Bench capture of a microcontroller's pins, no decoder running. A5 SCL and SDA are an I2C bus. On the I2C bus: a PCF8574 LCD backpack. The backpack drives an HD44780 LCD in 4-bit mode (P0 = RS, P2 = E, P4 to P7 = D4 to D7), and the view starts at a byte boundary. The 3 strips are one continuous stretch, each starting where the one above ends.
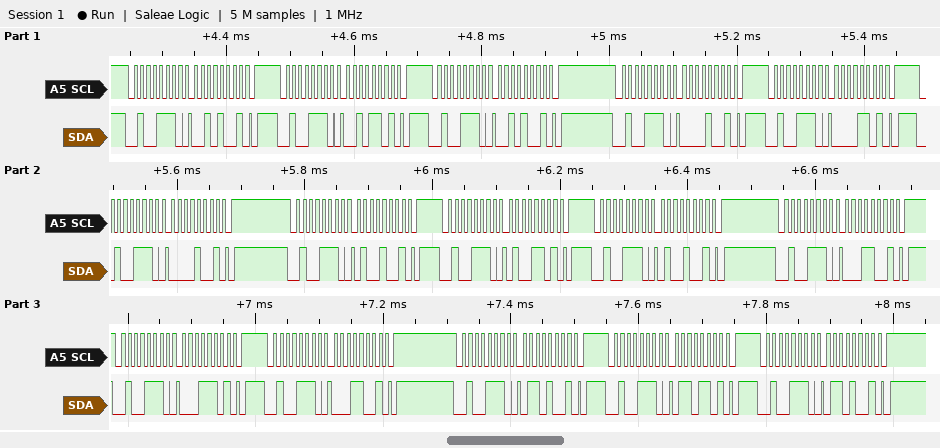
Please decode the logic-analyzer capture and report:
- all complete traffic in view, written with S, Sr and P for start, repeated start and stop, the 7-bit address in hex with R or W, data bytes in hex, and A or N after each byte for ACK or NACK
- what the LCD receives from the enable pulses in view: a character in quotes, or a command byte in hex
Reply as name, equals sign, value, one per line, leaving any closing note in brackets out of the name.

all complete traffic in view, written with S, Sr and P for start, repeated start and stop, the 7-bit address in hex with R or W, data bytes in hex, and A or N after each byte for ACK or NACK = S 27W A 29 A P S 27W A 2D A P S 27W A 29 A P S 27W A 09 A P S 27W A 0D A P S 27W A 09 A P S 27W A 49 A P S 27W A 4D A P S 27W A 49 A P S 27W A 19 A P S 27W A 1D A P S 27W A 19 A P S 27W A 69 A P S 27W A 6D A P S 27W A 69 A P
what the LCD receives from the enable pulses in view: a character in quotes, or a command byte in hex = ' ' 'A'
